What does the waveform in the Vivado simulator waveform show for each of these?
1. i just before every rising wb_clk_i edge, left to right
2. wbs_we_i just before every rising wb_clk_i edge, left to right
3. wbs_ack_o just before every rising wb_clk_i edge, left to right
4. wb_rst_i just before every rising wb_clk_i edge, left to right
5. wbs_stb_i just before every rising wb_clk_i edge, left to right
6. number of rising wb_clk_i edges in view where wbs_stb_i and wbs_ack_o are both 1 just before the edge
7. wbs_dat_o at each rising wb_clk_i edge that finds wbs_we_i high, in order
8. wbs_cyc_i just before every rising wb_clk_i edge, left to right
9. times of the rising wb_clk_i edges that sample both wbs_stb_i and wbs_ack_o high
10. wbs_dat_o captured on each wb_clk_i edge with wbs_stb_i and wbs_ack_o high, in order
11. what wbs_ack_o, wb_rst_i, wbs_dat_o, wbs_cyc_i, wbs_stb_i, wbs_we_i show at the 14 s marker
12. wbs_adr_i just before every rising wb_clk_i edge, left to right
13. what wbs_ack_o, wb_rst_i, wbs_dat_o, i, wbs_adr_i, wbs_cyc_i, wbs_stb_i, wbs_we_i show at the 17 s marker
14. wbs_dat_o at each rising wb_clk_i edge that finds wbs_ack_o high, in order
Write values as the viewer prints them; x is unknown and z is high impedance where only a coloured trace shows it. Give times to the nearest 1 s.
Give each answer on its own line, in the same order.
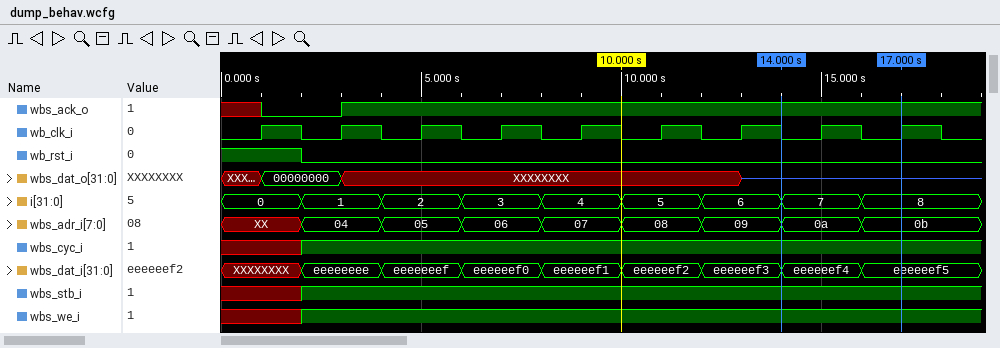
0, 1, 2, 3, 4, 5, 6, 7, 8
x 1 1 1 1 1 1 1 1
x 0 1 1 1 1 1 1 1
1 0 0 0 0 0 0 0 0
x 1 1 1 1 1 1 1 1
7
00000000, XXXXXXXX, XXXXXXXX, XXXXXXXX, XXXXXXXX, XXXXXXXX, z, z
x 1 1 1 1 1 1 1 1
5 s, 7 s, 9 s, 11 s, 13 s, 15 s, 17 s
XXXXXXXX, XXXXXXXX, XXXXXXXX, XXXXXXXX, XXXXXXXX, z, z
wbs_ack_o=1, wb_rst_i=0, wbs_dat_o=z, wbs_cyc_i=1, wbs_stb_i=1, wbs_we_i=1
XX, 04, 05, 06, 07, 08, 09, 0a, 0b
wbs_ack_o=1, wb_rst_i=0, wbs_dat_o=z, i=8, wbs_adr_i=0b, wbs_cyc_i=1, wbs_stb_i=1, wbs_we_i=1
XXXXXXXX, XXXXXXXX, XXXXXXXX, XXXXXXXX, XXXXXXXX, z, z
